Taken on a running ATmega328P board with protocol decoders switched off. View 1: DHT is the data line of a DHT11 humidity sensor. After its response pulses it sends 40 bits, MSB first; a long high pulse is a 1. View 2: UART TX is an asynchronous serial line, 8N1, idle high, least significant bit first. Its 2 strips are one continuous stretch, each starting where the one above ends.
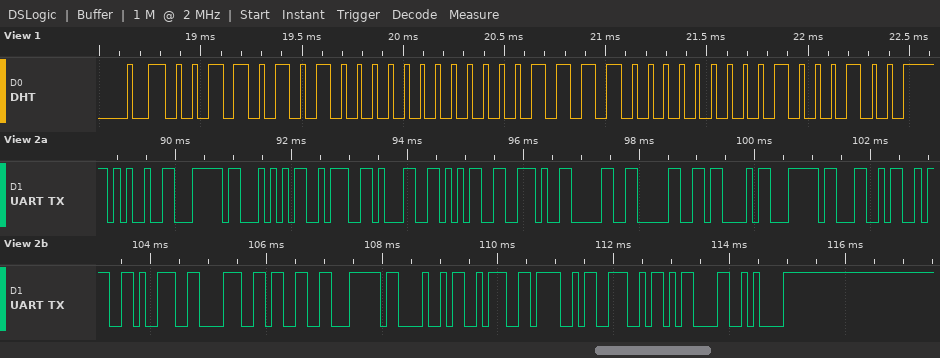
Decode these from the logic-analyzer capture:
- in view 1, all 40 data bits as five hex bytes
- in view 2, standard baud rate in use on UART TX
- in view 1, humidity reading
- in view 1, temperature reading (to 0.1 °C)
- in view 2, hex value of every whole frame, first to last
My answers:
35 00 0F 00 44
9600 baud
53 %
15.0 °C
25 7C 54 3A 31 35 2E 30 30 43 7C 4C 3A 39 38 33 7C 48 3A 4F 4E 0D 0A
